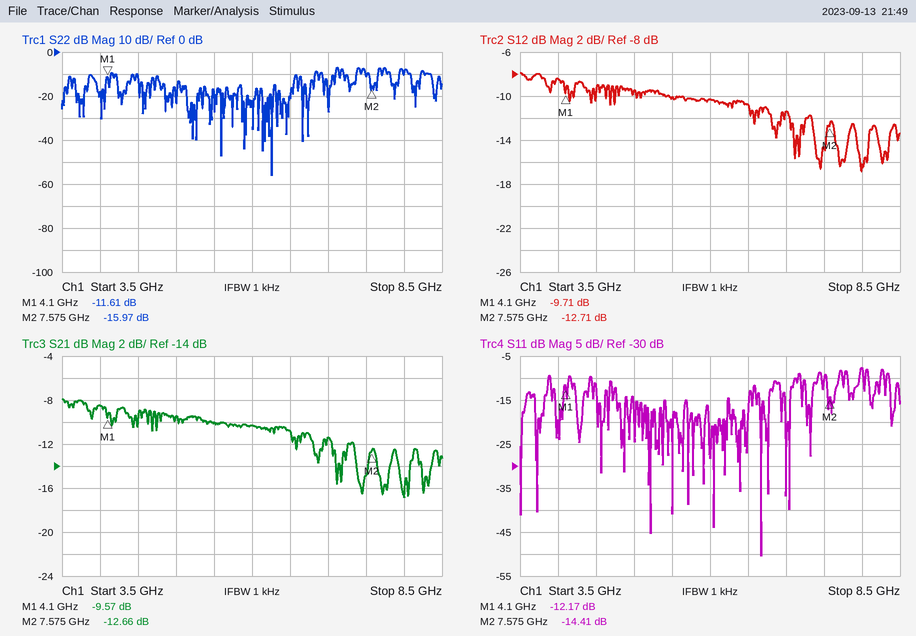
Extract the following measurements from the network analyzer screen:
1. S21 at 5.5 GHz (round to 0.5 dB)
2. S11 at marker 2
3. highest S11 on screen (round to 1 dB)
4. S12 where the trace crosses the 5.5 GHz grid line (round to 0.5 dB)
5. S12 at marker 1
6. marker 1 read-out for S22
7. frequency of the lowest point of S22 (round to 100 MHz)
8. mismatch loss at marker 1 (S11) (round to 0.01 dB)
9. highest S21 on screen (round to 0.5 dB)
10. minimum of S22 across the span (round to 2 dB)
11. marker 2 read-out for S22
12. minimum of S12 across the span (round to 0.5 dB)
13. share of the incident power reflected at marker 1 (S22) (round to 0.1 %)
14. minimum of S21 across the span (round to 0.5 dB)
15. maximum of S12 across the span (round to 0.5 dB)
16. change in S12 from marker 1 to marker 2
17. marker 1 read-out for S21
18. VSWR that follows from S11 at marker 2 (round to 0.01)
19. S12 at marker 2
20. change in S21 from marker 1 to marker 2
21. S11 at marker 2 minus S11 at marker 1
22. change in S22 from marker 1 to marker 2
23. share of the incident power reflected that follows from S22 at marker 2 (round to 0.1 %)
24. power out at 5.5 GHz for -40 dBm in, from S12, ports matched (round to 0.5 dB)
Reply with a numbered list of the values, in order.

1. -10.0 dB
2. -14.41 dB
3. -8 dB
4. -10.0 dB
5. -9.71 dB
6. -11.61 dB
7. 6.3 GHz
8. 0.27 dB
9. -8.0 dB
10. -56 dB
11. -15.97 dB
12. -17.0 dB
13. 6.9 %
14. -17.0 dB
15. -8.0 dB
16. -3.00 dB
17. -9.57 dB
18. 1.47
19. -12.71 dB
20. -3.09 dB
21. -2.24 dB
22. -4.36 dB
23. 2.5 %
24. -50.0 dBm
